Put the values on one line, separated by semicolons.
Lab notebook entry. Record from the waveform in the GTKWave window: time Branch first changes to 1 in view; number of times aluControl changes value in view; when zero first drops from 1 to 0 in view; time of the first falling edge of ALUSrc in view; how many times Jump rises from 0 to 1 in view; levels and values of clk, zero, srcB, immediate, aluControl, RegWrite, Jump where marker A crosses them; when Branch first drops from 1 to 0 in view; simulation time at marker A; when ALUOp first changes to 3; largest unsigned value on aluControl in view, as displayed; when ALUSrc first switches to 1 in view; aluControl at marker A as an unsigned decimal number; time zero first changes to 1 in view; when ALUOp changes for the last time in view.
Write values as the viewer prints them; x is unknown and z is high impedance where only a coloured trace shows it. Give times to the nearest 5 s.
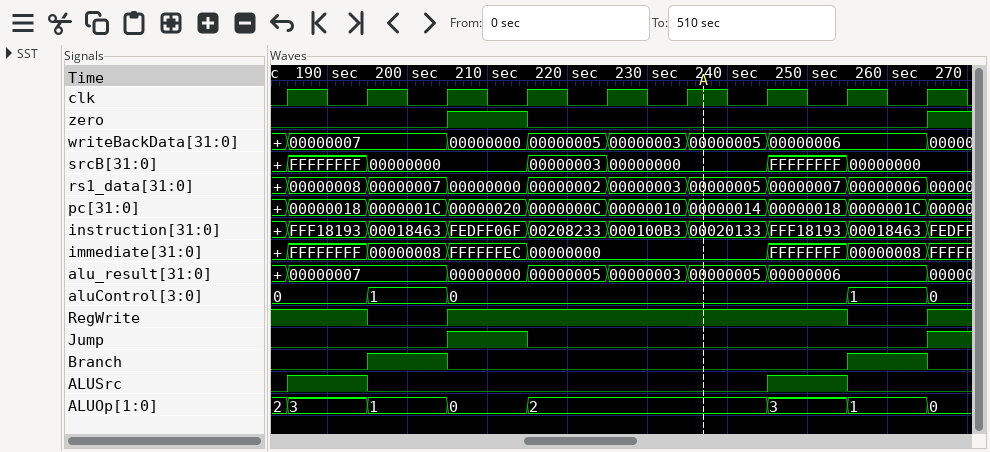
195 s; 4; 215 s; 195 s; 2; clk=1, zero=0, srcB=00000000, immediate=00000000, aluControl=0, RegWrite=1, Jump=0; 205 s; 235 s; 185 s; 1; 185 s; 0; 205 s; 265 s
